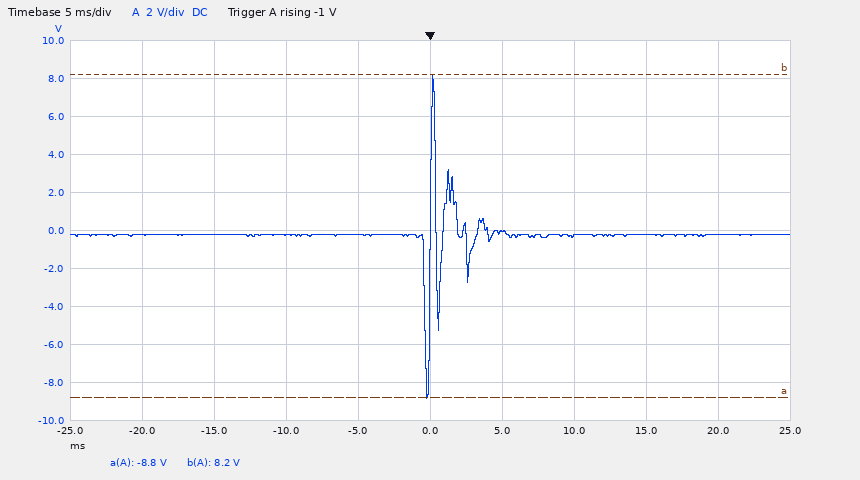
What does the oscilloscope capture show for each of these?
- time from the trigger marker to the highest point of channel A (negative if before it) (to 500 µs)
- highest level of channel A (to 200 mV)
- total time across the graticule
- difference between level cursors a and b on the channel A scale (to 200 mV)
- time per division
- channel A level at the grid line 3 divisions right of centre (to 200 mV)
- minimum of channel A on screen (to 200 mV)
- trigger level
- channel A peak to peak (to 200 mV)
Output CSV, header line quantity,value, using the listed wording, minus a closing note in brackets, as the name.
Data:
quantity,value
time from the trigger marker to the highest point of channel A (negative if before it),0.0 ms
highest level of channel A,8.2 V
total time across the graticule,50 ms
difference between level cursors a and b on the channel A scale,17.0 V
time per division,5 ms
channel A level at the grid line 3 divisions right of centre,-200 mV
minimum of channel A on screen,-8.8 V
trigger level,-1 V
channel A peak to peak,17.0 V
